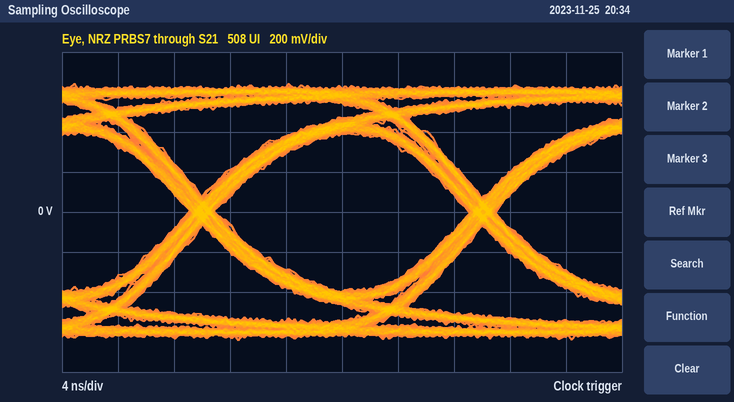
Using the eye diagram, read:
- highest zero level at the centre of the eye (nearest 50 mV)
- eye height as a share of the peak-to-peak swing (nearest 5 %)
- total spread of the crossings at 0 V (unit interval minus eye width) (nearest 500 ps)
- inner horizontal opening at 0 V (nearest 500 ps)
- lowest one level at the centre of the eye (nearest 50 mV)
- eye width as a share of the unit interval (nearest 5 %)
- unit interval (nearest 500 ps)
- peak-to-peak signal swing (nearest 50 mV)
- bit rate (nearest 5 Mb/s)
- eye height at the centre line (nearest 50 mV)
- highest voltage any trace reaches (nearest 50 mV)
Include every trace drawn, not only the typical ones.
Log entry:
-400 mV
60 %
2.0 ns
18.0 ns
400 mV
90 %
20.0 ns
1.30 V
50 Mb/s
800 mV
650 mV
